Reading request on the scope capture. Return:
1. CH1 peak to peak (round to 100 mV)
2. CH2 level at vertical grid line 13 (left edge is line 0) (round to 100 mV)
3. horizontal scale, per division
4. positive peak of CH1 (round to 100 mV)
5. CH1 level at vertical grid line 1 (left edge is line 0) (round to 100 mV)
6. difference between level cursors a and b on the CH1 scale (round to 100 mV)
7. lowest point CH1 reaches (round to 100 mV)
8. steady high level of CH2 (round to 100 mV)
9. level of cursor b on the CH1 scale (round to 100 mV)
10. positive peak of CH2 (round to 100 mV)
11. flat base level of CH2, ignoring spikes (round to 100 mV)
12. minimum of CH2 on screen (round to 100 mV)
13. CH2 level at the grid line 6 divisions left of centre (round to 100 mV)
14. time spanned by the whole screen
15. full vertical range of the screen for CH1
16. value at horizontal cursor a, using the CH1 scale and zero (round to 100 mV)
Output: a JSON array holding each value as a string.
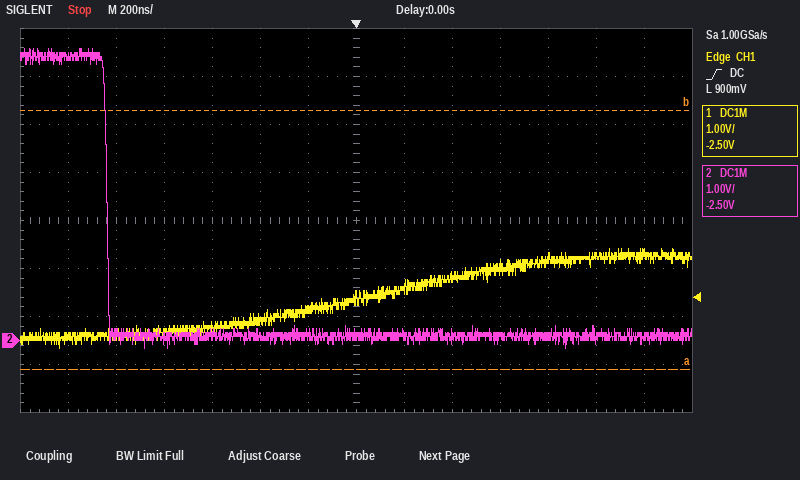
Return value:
["2.1 V", "100 mV", "200 ns", "1.9 V", "100 mV", "5.4 V", "-200 mV", "5.9 V", "4.8 V", "6.1 V", "100 mV", "-200 mV", "5.9 V", "2.8 µs", "8 V", "-600 mV"]
